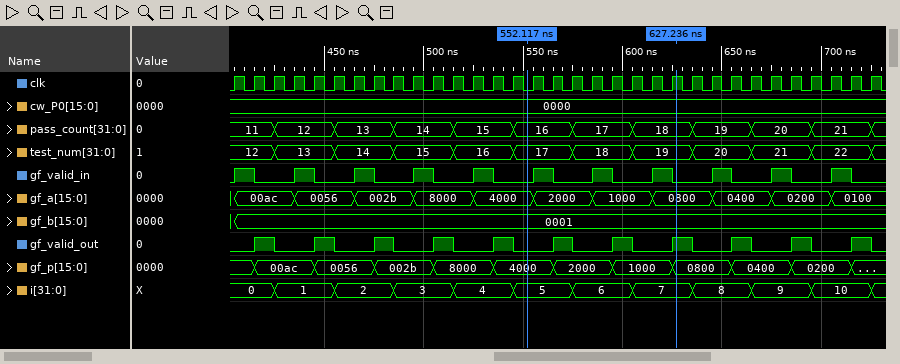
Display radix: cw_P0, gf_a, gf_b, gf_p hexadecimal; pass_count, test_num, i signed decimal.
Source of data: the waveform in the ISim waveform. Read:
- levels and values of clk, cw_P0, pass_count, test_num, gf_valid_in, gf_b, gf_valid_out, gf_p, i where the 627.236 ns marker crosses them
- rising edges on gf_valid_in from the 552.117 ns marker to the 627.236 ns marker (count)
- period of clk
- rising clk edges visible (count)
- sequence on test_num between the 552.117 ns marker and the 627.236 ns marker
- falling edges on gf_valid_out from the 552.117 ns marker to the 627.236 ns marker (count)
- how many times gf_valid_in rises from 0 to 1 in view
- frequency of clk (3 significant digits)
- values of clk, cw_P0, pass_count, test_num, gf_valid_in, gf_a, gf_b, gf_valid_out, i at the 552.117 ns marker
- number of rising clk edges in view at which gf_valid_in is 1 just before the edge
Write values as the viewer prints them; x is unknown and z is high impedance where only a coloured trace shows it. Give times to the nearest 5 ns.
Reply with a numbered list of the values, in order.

1. clk=1, cw_P0=0000, pass_count=18, test_num=19, gf_valid_in=0, gf_b=0001, gf_valid_out=1, gf_p=0800, i=7
2. 3
3. 10 ns
4. 33
5. 17, 18, 19
6. 2
7. 11
8. 100 MHz
9. clk=0, cw_P0=0000, pass_count=16, test_num=17, gf_valid_in=0, gf_a=4000, gf_b=0001, gf_valid_out=0, i=5
10. 11
